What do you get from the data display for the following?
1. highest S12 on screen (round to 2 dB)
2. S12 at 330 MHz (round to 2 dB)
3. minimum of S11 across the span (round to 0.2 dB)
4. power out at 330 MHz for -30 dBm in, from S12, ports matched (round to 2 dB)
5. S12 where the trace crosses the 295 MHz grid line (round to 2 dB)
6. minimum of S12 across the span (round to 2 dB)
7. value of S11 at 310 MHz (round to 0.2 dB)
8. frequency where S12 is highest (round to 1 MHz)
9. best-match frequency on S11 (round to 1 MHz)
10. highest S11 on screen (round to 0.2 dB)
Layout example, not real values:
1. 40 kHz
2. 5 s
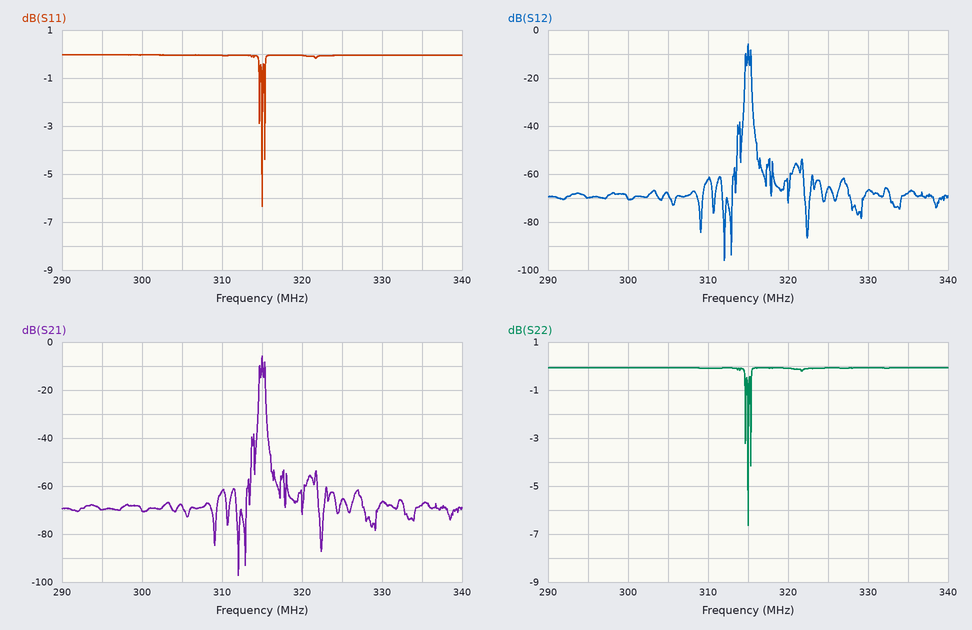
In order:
1. -6 dB
2. -66 dB
3. -6.4 dB
4. -96 dBm
5. -70 dB
6. -96 dB
7. 0.0 dB
8. 315 MHz
9. 315 MHz
10. 0.0 dB
